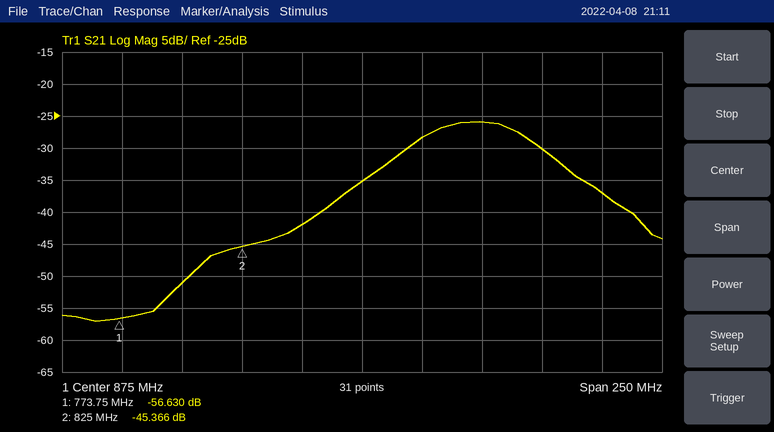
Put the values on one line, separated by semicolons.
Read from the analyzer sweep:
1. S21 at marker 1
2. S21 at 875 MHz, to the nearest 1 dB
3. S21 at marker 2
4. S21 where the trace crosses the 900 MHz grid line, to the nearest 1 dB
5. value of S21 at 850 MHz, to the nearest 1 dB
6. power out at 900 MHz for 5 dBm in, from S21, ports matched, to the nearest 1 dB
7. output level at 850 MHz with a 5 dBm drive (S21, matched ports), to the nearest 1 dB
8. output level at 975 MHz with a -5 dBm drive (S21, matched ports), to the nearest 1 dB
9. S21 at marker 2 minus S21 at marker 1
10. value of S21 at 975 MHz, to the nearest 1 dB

-56.630 dB; -35 dB; -45.366 dB; -28 dB; -42 dB; -23 dBm; -37 dBm; -42 dBm; 11.264 dB; -37 dB
